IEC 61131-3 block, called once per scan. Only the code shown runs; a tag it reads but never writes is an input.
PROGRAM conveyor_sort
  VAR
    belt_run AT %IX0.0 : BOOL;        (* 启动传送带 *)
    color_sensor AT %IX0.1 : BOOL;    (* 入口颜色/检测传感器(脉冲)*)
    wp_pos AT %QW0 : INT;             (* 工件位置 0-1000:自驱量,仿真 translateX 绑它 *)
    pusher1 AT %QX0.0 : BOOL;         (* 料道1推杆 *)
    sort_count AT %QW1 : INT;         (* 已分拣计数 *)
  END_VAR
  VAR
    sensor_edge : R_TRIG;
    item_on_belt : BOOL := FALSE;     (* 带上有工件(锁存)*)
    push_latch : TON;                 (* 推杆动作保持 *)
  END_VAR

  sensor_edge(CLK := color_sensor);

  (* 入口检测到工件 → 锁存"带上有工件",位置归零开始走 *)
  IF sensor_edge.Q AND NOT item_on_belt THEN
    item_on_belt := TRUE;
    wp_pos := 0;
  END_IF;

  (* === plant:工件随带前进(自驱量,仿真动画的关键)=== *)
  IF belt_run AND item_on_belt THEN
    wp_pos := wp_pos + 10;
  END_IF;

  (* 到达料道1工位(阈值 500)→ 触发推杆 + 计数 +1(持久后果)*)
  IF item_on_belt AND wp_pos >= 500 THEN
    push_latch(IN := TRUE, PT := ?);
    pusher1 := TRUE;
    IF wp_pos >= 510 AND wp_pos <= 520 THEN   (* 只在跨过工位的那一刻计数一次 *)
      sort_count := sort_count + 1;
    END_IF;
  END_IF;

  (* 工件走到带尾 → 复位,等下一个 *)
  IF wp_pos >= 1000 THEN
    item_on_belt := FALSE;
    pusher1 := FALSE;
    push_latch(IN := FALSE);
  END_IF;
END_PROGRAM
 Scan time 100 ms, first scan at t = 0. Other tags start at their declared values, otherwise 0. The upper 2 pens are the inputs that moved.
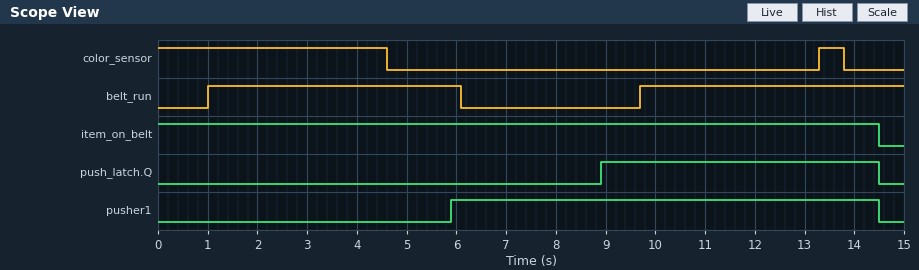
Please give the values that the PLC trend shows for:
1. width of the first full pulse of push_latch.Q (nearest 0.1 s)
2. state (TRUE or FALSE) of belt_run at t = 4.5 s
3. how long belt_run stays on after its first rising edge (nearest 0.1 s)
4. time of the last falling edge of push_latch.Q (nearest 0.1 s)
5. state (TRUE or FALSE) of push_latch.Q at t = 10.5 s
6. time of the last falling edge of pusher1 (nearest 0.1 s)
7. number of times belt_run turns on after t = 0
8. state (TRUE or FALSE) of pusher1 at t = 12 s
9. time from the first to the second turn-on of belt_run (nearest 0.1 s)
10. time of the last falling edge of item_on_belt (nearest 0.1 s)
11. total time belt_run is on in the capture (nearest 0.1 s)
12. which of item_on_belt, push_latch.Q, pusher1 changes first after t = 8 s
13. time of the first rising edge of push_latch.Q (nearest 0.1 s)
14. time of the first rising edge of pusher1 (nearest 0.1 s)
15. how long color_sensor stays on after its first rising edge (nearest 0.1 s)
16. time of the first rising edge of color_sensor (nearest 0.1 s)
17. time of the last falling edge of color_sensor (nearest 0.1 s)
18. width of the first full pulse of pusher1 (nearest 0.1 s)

5.6 s
TRUE
5.1 s
14.5 s
TRUE
14.5 s
2
TRUE
8.7 s
14.5 s
10.4 s
push_latch.Q
8.9 s
5.9 s
0.5 s
13.3 s
13.8 s
8.6 s
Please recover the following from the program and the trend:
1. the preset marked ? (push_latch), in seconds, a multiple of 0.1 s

3.0 s
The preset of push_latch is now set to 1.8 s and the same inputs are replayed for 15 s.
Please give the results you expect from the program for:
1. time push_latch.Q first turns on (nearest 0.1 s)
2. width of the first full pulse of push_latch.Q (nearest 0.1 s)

7.7 s
6.8 s
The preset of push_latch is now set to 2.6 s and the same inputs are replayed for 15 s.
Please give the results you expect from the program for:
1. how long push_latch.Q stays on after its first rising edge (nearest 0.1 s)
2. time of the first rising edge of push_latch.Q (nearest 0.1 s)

6.0 s
8.5 s
